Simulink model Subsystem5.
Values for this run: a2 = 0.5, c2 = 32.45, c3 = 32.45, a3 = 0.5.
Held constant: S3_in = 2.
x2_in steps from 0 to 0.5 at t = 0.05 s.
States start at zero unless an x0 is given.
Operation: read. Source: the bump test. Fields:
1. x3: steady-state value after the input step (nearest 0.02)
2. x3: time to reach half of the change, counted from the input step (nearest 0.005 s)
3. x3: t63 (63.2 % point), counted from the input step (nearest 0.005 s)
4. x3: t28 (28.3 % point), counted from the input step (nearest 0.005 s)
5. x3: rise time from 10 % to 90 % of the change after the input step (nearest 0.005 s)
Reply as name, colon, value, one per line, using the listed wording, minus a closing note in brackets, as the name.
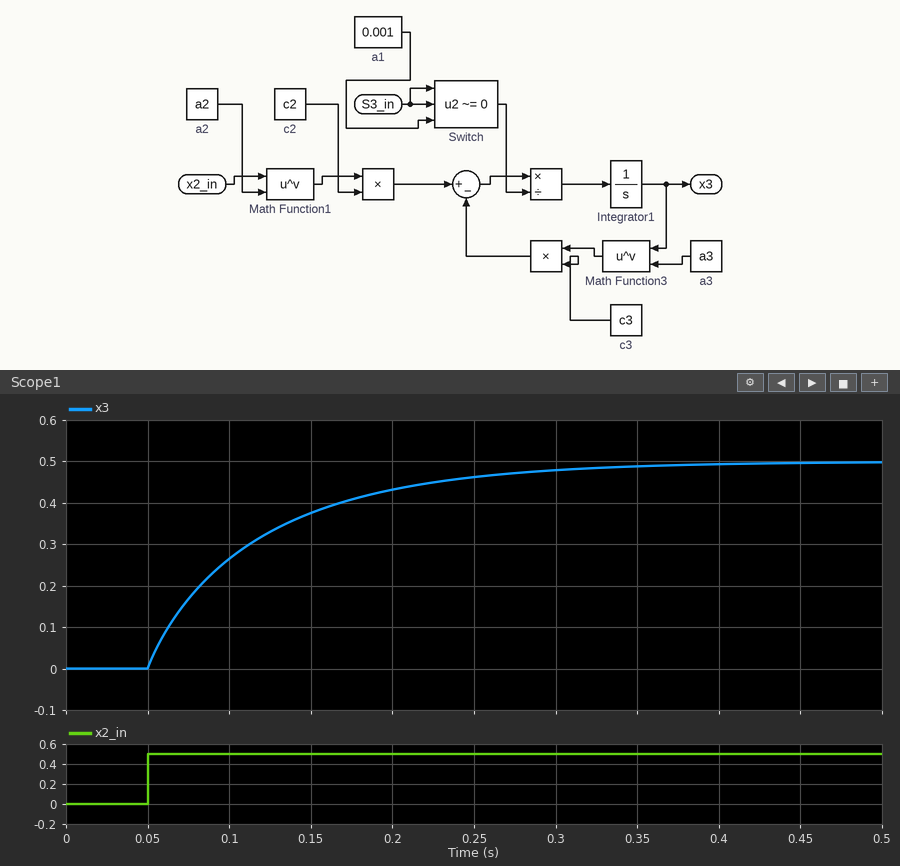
x3: steady-state value after the input step: 0.50
x3: time to reach half of the change, counted from the input step: 0.045 s
x3: t63 (63.2 % point), counted from the input step: 0.070 s
x3: t28 (28.3 % point), counted from the input step: 0.020 s
x3: rise time from 10 % to 90 % of the change after the input step: 0.170 s
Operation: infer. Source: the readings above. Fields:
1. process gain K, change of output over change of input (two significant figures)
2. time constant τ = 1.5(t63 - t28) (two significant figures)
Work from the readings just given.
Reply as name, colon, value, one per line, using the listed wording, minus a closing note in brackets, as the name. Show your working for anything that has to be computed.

process gain K, change of output over change of input: (0.5 - 0) / 0.5 = 1.0
time constant τ = 1.5(t63 - t28): 1.5 × (0.07 - 0.02) = 0.075 s
